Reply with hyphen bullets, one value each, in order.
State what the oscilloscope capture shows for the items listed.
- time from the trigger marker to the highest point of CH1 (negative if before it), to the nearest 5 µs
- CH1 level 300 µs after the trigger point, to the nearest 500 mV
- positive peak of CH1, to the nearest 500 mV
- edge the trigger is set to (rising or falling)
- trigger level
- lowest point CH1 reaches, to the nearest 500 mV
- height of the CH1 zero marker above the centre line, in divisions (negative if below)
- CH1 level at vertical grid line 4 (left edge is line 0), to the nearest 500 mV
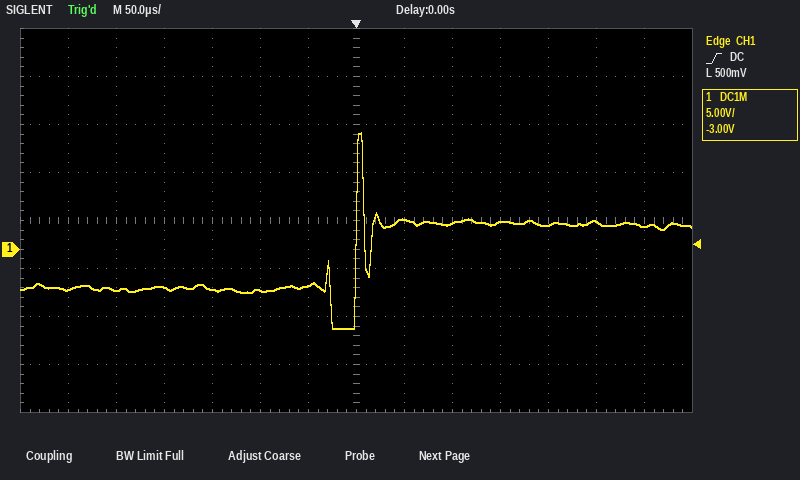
- +5 µs
- 2.5 V
- 12.0 V
- rising
- 500 mV
- -8.0 V
- -0.6 div
- -4.0 V
